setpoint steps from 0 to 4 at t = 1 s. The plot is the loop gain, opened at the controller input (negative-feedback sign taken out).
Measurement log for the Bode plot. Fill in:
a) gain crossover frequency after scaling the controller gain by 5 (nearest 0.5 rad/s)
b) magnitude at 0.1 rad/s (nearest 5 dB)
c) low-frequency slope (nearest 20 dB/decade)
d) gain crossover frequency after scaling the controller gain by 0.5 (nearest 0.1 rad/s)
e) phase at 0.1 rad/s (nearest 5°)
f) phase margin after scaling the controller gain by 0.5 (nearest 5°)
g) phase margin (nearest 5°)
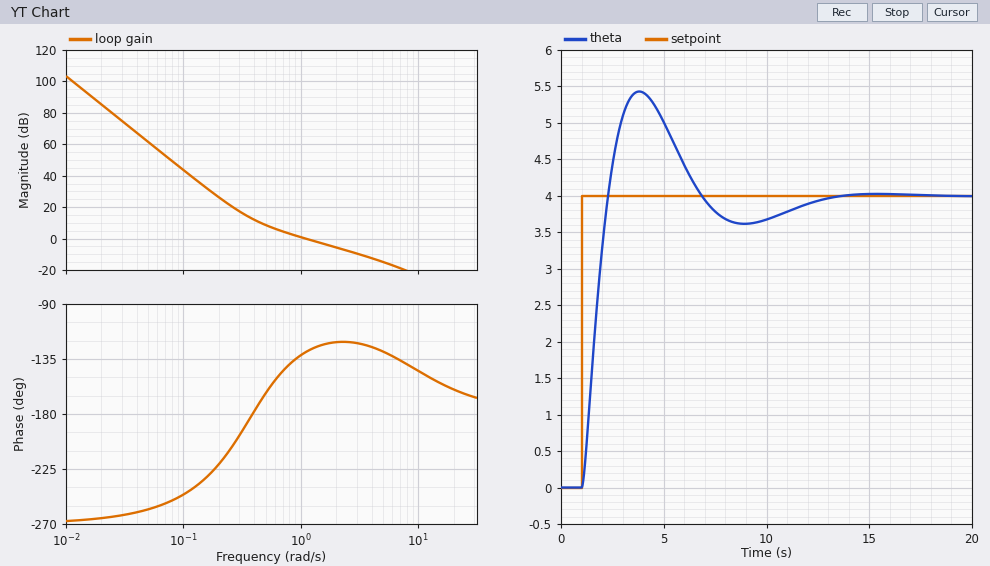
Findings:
4.5 rad/s
45 dB
-60 dB/decade
0.6 rad/s
-245°
30°
50°
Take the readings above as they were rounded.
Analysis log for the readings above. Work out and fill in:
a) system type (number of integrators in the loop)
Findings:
3
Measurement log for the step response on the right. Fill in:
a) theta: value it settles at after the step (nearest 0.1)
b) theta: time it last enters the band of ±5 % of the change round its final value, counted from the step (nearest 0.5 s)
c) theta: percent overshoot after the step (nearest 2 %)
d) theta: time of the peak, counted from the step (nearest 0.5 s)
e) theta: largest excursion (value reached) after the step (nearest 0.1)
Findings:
4.0
10.0 s
36 %
3.0 s
5.4
